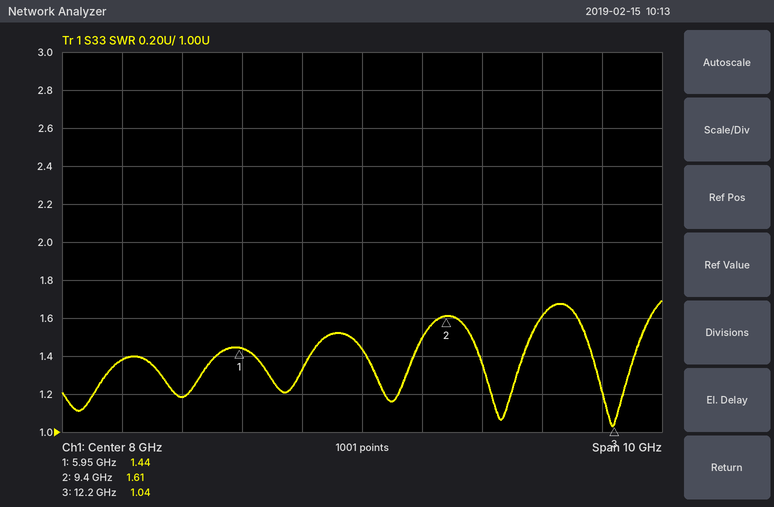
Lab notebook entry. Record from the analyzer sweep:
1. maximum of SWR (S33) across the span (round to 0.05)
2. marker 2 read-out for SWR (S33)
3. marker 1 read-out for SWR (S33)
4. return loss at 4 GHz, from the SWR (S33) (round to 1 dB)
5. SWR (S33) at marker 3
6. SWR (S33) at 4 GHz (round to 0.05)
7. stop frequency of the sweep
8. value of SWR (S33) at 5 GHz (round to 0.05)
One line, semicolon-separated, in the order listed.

1.70; 1.61; 1.44; 16 dB; 1.04; 1.40; 13 GHz; 1.20
